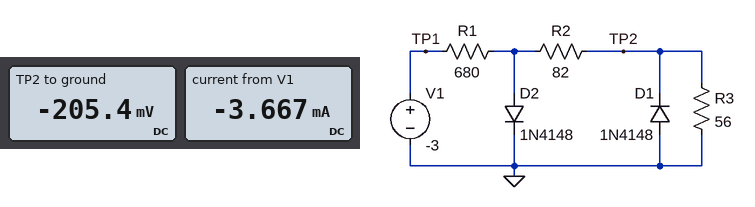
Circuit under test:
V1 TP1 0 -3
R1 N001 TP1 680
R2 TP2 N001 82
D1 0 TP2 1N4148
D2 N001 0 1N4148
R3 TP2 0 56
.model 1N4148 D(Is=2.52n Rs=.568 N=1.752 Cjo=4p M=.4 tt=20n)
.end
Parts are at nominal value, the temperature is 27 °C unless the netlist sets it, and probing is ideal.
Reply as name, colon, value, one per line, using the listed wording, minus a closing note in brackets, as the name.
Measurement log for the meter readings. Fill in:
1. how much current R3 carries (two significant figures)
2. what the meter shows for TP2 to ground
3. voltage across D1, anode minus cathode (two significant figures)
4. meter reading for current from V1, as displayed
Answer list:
how much current R3 carries: 3.7 mA
what the meter shows for TP2 to ground: -205.4 mV
voltage across D1, anode minus cathode: 210 mV
meter reading for current from V1, as displayed: -3.667 mA
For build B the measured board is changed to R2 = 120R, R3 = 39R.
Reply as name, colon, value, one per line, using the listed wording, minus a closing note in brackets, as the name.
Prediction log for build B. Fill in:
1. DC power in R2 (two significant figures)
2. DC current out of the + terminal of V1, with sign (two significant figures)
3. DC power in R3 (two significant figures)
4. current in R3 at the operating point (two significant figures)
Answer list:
DC power in R2: 1.5 mW
DC current out of the + terminal of V1, with sign: -3.6 mA
DC power in R3: 500 µW
current in R3 at the operating point: 3.6 mA
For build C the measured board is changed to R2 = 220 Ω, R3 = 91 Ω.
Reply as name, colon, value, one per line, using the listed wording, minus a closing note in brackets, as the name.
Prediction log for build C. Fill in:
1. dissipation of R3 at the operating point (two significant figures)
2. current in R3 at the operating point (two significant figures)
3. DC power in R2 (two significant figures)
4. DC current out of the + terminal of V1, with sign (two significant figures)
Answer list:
dissipation of R3 at the operating point: 830 µW
current in R3 at the operating point: 3.0 mA
DC power in R2: 2.0 mW
DC current out of the + terminal of V1, with sign: -3.0 mA
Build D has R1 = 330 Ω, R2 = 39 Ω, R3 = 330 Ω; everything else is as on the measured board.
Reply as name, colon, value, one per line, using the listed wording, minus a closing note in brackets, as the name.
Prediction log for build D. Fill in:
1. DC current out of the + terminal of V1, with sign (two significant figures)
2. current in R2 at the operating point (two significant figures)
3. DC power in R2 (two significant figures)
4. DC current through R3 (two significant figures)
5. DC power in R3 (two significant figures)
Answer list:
DC current out of the + terminal of V1, with sign: -6.4 mA
current in R2 at the operating point: 6.4 mA
DC power in R2: 1.6 mW
DC current through R3: 2.0 mA
DC power in R3: 1.3 mW
